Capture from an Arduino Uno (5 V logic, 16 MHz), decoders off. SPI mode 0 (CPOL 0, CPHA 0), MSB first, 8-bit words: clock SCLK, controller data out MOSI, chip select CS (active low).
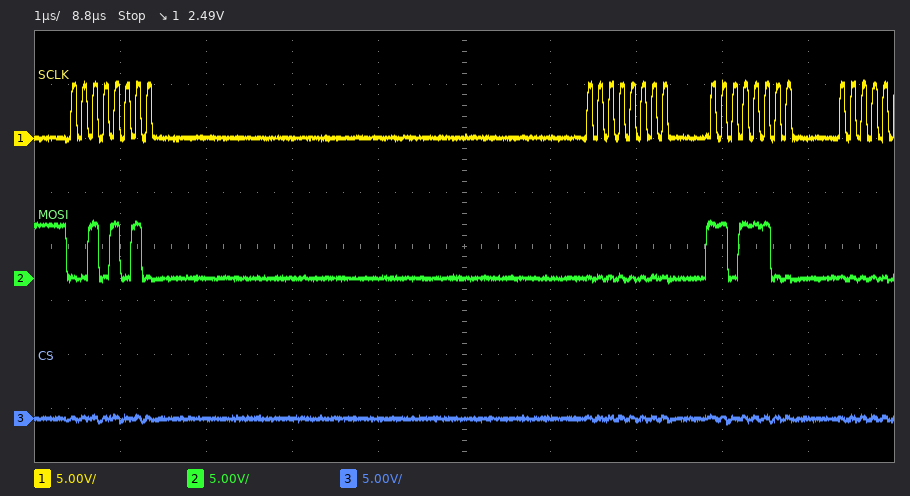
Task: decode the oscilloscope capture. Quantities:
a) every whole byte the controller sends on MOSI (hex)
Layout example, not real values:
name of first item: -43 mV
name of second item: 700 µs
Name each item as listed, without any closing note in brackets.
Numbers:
every whole byte the controller sends on MOSI: 0x2A 0x00 0xDC
